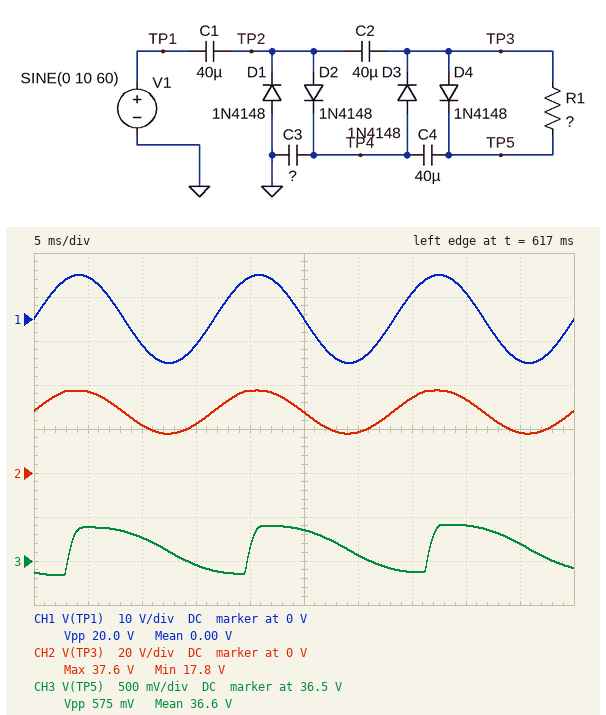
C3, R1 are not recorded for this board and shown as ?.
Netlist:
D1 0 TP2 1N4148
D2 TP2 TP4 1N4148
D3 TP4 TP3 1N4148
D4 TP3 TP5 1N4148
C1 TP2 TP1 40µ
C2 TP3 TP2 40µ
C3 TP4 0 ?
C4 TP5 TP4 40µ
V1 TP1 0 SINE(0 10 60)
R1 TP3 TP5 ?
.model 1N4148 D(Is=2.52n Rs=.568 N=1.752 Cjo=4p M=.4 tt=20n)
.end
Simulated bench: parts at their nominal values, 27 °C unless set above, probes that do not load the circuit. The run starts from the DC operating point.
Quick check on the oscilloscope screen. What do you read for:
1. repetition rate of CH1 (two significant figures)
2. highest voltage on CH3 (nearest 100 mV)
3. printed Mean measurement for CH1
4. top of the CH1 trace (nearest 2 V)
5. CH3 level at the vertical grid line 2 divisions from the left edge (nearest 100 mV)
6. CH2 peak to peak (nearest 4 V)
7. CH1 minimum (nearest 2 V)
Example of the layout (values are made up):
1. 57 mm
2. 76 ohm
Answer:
1. 60 Hz
2. 36.9 V
3. 0.00 V
4. 10 V
5. 36.8 V
6. 20 V
7. -10 V
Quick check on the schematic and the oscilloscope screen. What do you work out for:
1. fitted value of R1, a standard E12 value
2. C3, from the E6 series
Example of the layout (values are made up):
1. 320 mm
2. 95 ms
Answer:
1. 10 kΩ
2. 100 µF
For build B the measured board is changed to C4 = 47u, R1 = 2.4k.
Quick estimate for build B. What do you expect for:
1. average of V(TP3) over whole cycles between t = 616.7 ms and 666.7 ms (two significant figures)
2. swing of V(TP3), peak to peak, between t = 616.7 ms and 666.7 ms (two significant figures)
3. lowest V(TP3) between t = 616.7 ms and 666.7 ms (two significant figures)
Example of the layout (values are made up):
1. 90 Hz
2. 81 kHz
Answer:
1. 27 V
2. 19 V
3. 17 V
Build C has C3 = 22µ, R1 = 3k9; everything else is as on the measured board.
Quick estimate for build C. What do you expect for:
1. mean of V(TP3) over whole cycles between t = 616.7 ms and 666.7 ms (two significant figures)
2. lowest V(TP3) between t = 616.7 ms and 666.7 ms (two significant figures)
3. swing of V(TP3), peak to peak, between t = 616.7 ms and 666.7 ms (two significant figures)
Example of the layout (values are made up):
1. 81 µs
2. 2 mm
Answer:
1. 27 V
2. 17 V
3. 19 V
